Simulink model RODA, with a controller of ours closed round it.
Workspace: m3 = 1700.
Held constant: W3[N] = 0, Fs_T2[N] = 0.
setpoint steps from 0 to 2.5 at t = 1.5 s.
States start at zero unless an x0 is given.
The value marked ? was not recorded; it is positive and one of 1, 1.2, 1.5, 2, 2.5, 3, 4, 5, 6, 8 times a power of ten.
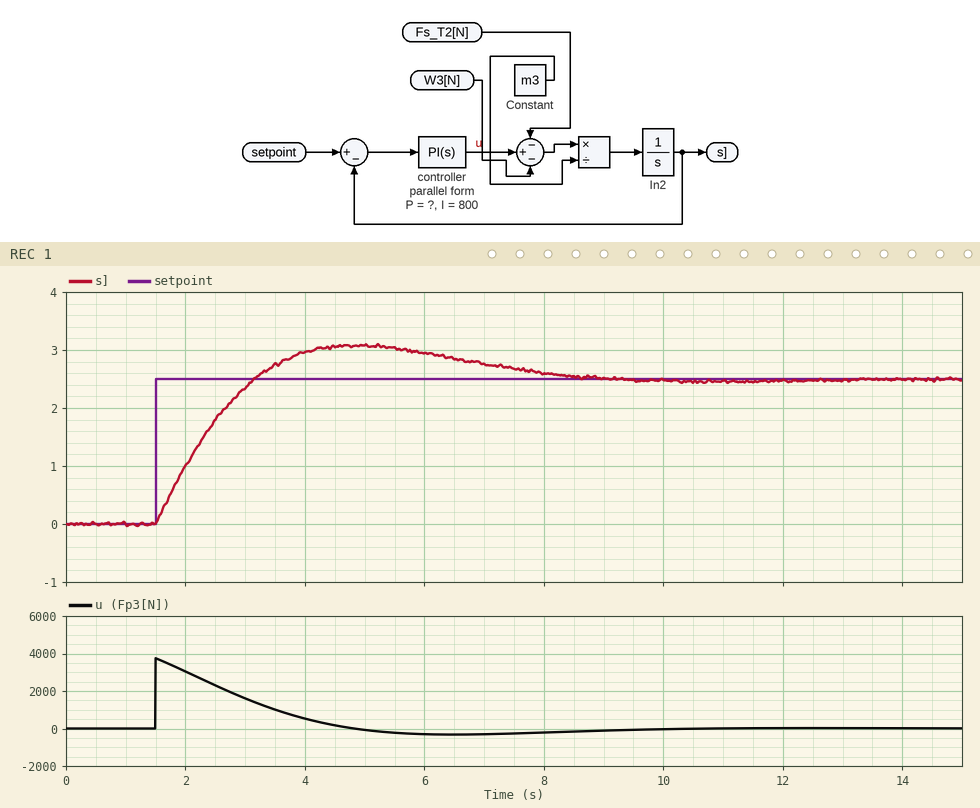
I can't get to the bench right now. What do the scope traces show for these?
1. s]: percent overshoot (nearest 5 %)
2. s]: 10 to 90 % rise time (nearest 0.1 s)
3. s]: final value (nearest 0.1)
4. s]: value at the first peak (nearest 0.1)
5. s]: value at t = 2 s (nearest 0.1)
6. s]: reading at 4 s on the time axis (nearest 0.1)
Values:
25 %
1.3 s
2.5
3.1
1.0
3.0
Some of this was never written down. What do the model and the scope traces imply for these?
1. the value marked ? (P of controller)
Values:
1500
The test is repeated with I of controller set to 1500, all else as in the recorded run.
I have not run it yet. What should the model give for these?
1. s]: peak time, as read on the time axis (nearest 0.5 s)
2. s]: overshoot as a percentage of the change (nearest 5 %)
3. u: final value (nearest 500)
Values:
4.0 s
30 %
0
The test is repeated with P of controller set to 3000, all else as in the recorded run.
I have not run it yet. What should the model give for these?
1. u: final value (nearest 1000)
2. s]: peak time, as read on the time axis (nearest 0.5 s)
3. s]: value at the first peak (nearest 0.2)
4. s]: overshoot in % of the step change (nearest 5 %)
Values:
0
4.0 s
2.8
10 %
